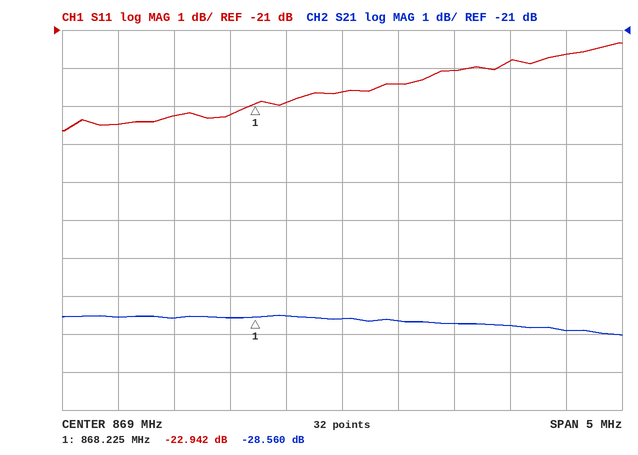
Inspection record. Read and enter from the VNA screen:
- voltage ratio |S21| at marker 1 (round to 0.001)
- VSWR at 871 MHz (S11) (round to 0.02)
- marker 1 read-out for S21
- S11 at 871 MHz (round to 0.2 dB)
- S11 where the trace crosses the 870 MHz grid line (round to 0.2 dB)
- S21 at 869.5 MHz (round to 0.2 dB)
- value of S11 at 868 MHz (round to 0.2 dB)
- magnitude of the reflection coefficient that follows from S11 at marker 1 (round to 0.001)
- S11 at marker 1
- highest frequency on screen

0.037
1.18
-28.560 dB
-21.6 dB
-22.0 dB
-28.6 dB
-23.2 dB
0.071
-22.942 dB
871.5 MHz
